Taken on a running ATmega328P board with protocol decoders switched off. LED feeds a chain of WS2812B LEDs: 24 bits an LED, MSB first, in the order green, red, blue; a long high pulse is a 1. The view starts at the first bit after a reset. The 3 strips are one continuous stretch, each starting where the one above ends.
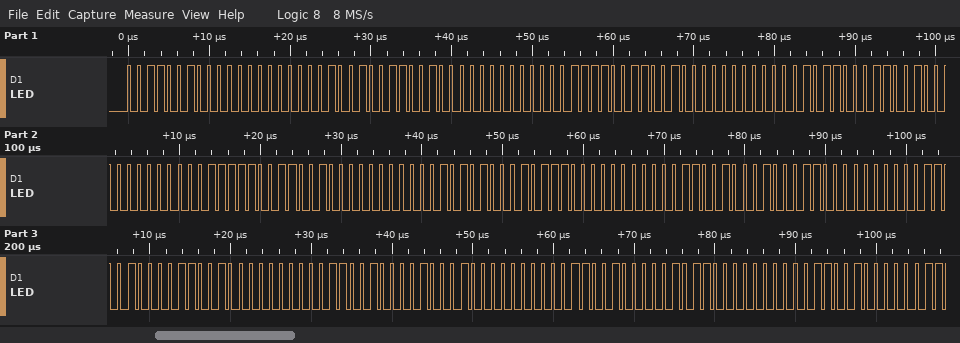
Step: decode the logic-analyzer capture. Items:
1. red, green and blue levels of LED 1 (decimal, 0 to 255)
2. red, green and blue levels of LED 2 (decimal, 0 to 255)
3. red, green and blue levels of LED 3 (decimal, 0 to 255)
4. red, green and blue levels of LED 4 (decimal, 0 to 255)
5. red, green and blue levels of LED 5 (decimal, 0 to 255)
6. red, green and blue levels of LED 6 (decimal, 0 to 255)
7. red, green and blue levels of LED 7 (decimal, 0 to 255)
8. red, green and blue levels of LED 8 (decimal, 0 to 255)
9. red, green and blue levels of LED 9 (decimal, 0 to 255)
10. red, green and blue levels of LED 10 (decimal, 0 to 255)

0, 50, 9
0, 50, 15
0, 50, 22
0, 50, 31
0, 50, 42
0, 46, 50
0, 35, 50
0, 25, 50
0, 17, 50
0, 11, 50
